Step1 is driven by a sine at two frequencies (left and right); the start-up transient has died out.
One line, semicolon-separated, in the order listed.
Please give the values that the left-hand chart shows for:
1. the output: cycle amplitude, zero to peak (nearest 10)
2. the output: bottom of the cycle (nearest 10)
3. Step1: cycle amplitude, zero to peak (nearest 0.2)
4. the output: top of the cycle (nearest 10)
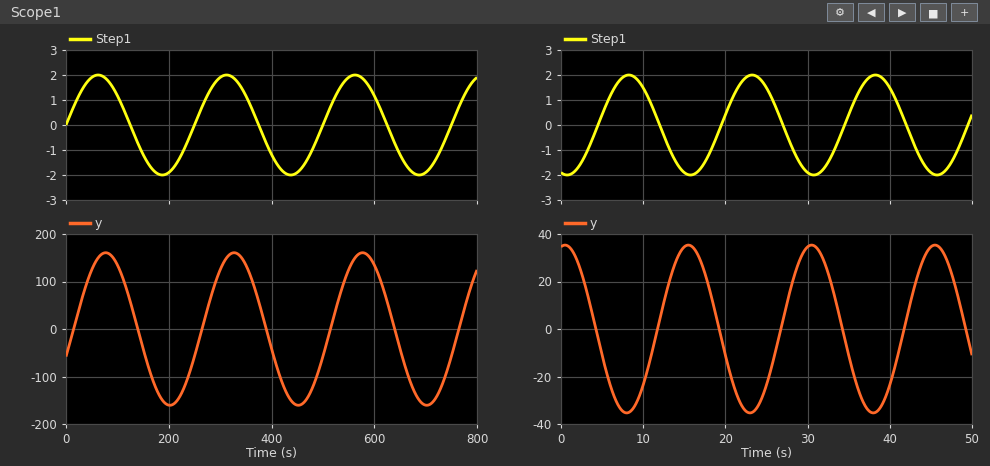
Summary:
160; -160; 2.0; 160
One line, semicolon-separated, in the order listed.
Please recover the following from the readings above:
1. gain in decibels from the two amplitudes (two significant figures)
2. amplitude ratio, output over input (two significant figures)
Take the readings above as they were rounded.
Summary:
38 dB; 80
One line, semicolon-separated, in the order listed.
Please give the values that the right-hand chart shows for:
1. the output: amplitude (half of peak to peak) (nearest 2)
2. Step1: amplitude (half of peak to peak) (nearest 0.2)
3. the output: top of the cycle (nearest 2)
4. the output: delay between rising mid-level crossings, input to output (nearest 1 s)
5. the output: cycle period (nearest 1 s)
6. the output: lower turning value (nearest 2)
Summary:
36; 2.0; 36; 7 s; 15 s; -36
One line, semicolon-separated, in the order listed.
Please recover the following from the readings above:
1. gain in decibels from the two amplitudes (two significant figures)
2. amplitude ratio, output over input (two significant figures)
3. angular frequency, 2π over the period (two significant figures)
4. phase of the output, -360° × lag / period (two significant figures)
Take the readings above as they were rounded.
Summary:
25 dB; 18; 0.42 rad/s; -170°
